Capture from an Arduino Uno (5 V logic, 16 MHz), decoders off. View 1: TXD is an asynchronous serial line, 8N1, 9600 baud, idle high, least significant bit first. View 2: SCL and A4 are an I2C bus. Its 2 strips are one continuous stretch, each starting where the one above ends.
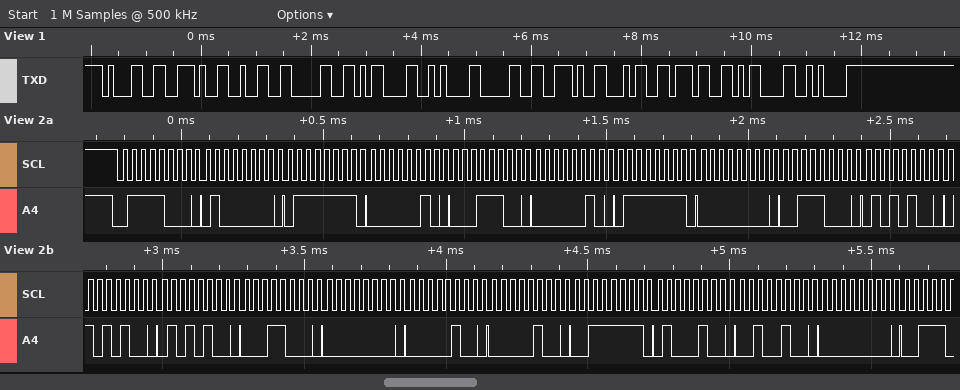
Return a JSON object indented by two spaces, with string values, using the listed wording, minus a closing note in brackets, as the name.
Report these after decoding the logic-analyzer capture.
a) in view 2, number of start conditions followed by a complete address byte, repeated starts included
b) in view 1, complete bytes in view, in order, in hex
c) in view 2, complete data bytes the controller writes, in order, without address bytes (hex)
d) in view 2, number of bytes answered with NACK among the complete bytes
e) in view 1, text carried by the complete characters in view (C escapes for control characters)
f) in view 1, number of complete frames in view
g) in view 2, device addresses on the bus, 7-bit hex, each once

{
  "in view 2, number of start conditions followed by a complete address byte, repeated starts included": "1",
  "in view 1, complete bytes in view, in order, in hex": "0x31 0x2E 0x32 0x30 0x0D 0x0A 0x30 0x2E 0x34 0x37 0x0D 0x0A",
  "in view 2, complete data bytes the controller writes, in order, without address bytes": "40 7F 02 1C 02 7F 00 38 54 54 54 18 00 04 04 3F 44 24 00",
  "in view 2, number of bytes answered with NACK among the complete bytes": "0",
  "in view 1, text carried by the complete characters in view": "\"1.20\\r\\n0.47\\r\\n\"",
  "in view 1, number of complete frames in view": "12",
  "in view 2, device addresses on the bus, 7-bit hex, each once": "0x3C"
}
